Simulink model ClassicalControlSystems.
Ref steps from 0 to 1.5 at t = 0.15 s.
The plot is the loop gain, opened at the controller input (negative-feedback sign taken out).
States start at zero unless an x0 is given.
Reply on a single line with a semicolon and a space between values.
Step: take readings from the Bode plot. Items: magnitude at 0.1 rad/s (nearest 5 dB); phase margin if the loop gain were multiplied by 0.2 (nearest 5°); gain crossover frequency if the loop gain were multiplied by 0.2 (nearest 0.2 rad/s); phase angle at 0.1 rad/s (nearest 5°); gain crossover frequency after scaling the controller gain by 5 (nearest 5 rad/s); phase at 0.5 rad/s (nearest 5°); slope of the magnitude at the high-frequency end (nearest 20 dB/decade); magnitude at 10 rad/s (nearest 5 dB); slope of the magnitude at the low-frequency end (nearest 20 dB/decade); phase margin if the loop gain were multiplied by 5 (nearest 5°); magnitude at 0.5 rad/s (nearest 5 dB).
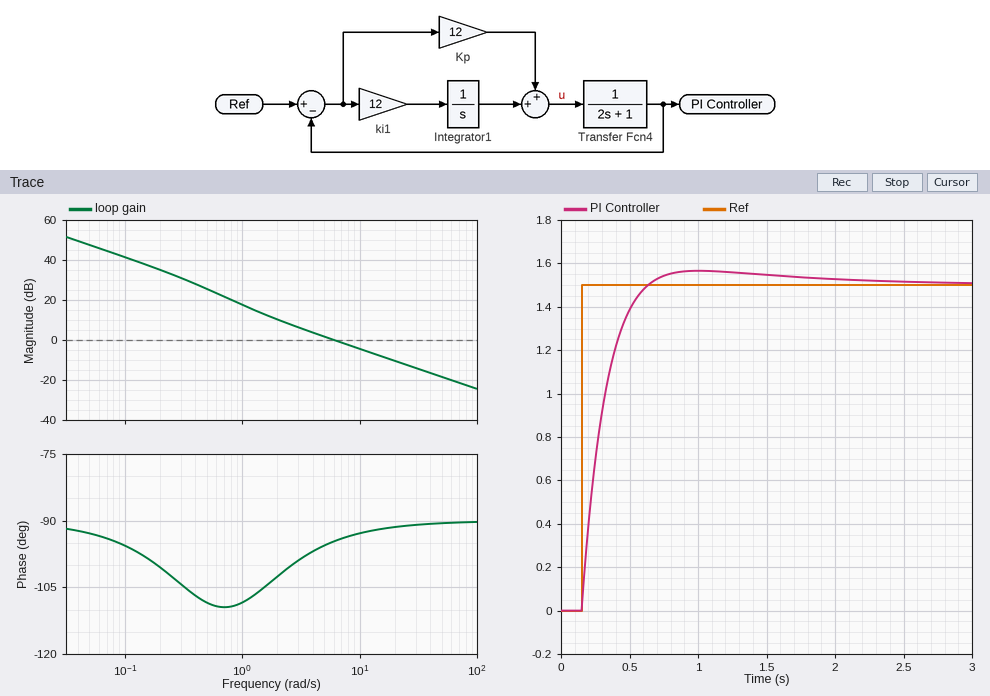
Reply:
40 dB; 75°; 1.4 rad/s; -95°; 30 rad/s; -110°; -20 dB/decade; -5 dB; -20 dB/decade; 90°; 25 dB
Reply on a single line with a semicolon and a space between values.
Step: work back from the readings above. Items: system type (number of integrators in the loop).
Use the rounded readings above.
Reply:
1
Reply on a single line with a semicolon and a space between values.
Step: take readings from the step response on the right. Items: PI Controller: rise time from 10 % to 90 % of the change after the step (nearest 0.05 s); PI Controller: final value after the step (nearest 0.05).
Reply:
0.30 s; 1.50
